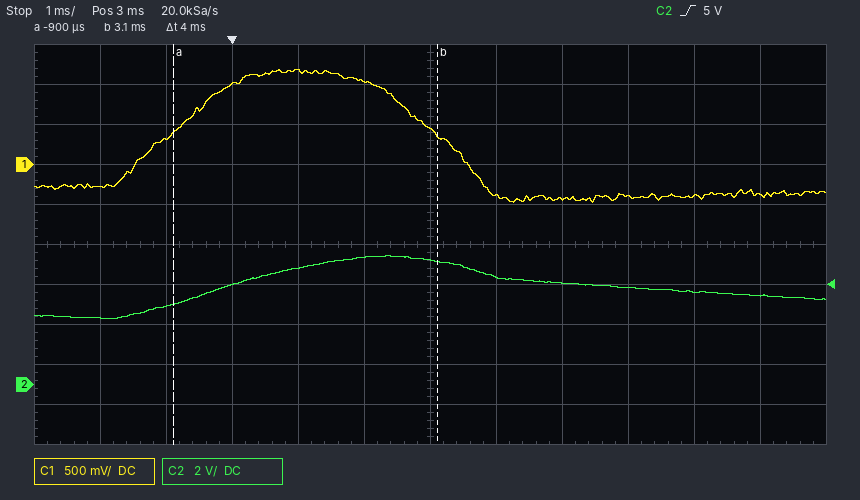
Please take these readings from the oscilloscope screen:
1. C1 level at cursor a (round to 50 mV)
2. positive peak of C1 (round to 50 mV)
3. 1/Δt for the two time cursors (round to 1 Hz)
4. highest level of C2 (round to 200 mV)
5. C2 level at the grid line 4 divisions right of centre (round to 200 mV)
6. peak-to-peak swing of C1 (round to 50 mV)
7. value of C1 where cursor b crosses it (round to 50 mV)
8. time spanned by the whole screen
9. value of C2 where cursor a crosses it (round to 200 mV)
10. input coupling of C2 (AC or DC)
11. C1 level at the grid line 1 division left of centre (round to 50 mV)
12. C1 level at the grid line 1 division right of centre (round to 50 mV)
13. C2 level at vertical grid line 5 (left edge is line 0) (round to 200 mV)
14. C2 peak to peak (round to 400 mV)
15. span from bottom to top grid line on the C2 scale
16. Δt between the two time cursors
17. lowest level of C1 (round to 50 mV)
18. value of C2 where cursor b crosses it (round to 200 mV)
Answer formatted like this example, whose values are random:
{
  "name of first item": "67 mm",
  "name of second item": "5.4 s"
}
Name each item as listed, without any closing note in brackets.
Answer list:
{
  "C1 level at cursor a": "400 mV",
  "positive peak of C1": "1.20 V",
  "1/Δt for the two time cursors": "250 Hz",
  "highest level of C2": "6.4 V",
  "C2 level at the grid line 4 divisions right of centre": "4.6 V",
  "peak-to-peak swing of C1": "1.65 V",
  "value of C1 where cursor b crosses it": "350 mV",
  "time spanned by the whole screen": "12 ms",
  "value of C2 where cursor a crosses it": "4.0 V",
  "input coupling of C2": "DC",
  "C1 level at the grid line 1 division left of centre": "1.05 V",
  "C1 level at the grid line 1 division right of centre": "-400 mV",
  "C2 level at vertical grid line 5 (left edge is line 0)": "6.4 V",
  "C2 peak to peak": "3.2 V",
  "span from bottom to top grid line on the C2 scale": "20 V",
  "Δt between the two time cursors": "4 ms",
  "lowest level of C1": "-450 mV",
  "value of C2 where cursor b crosses it": "6.2 V"
}
